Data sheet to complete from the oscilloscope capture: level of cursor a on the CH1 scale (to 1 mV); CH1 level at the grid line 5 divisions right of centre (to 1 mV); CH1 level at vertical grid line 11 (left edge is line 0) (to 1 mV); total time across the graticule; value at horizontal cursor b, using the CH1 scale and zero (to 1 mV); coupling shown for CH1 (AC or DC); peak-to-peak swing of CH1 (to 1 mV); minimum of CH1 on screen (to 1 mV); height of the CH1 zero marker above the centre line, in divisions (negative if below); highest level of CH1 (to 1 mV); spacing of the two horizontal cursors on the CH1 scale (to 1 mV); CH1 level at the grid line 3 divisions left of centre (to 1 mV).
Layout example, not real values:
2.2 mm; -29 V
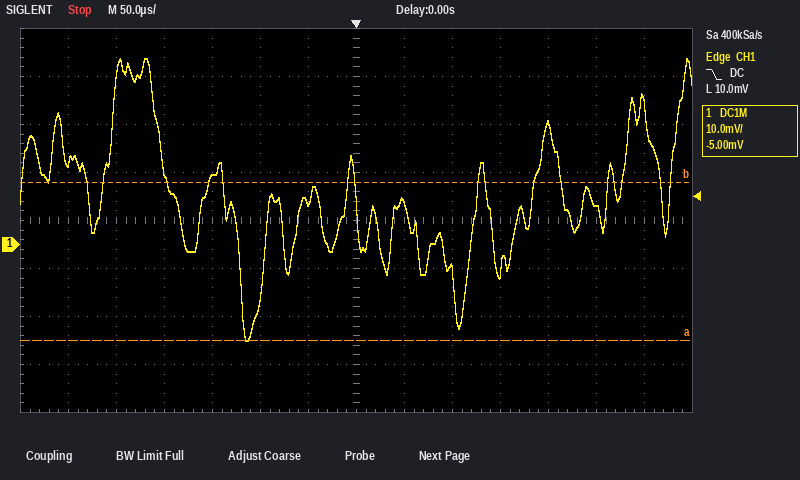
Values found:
-20 mV; 8 mV; 25 mV; 700 µs; 13 mV; DC; 59 mV; -20 mV; -0.5 div; 39 mV; 33 mV; 14 mV
